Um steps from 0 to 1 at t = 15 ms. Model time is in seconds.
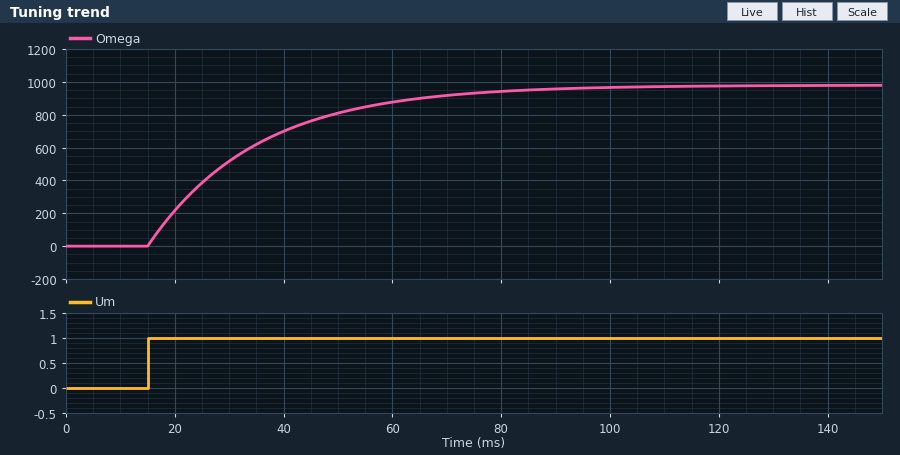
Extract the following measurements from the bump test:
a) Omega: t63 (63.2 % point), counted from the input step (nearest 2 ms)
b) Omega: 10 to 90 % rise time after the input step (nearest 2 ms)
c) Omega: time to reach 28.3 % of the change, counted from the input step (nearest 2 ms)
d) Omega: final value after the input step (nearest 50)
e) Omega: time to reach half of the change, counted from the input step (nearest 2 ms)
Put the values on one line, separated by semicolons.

20 ms; 44 ms; 6 ms; 1000; 14 ms
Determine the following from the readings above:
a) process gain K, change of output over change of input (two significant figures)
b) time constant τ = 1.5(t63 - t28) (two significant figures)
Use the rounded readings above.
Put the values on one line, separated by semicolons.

1000; 21 ms
